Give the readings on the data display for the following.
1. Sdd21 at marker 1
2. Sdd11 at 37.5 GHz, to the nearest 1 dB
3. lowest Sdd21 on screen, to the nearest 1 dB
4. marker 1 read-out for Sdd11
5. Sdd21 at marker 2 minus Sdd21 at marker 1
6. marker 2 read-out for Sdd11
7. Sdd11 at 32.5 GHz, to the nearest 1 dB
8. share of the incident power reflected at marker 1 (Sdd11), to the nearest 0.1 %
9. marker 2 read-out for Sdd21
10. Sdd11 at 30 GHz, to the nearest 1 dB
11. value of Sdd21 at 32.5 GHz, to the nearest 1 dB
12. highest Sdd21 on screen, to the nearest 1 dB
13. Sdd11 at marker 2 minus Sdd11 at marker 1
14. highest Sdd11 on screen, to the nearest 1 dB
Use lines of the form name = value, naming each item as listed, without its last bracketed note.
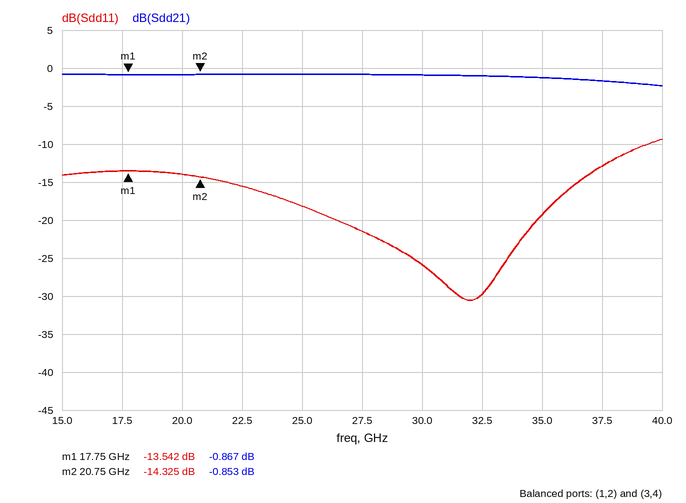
Sdd21 at marker 1 = -0.867 dB
Sdd11 at 37.5 GHz, to the nearest 1 dB = -13 dB
lowest Sdd21 on screen, to the nearest 1 dB = -2 dB
marker 1 read-out for Sdd11 = -13.542 dB
Sdd21 at marker 2 minus Sdd21 at marker 1 = 0.014 dB
marker 2 read-out for Sdd11 = -14.325 dB
Sdd11 at 32.5 GHz, to the nearest 1 dB = -30 dB
share of the incident power reflected at marker 1 (Sdd11), to the nearest 0.1 % = 4.4 %
marker 2 read-out for Sdd21 = -0.853 dB
Sdd11 at 30 GHz, to the nearest 1 dB = -26 dB
value of Sdd21 at 32.5 GHz, to the nearest 1 dB = -1 dB
highest Sdd21 on screen, to the nearest 1 dB = -1 dB
Sdd11 at marker 2 minus Sdd11 at marker 1 = -0.783 dB
highest Sdd11 on screen, to the nearest 1 dB = -9 dB
